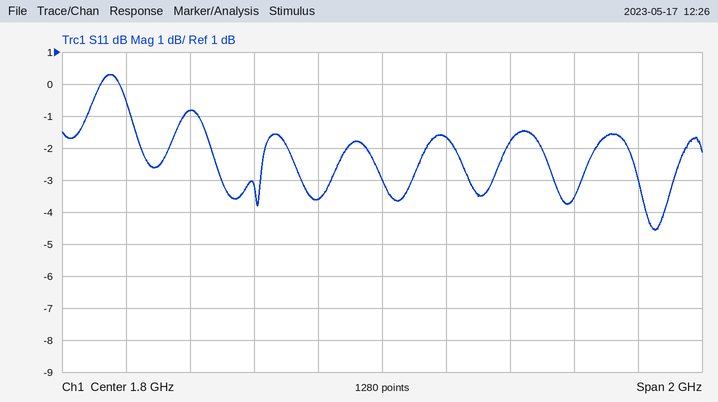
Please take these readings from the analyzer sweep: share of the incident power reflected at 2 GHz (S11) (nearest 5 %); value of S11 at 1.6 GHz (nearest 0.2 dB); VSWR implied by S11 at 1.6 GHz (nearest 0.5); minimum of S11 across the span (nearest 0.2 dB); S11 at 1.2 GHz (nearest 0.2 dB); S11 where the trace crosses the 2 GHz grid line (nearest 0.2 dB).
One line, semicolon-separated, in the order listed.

70 %; -3.6 dB; 5.0; -4.6 dB; -0.8 dB; -1.6 dB
